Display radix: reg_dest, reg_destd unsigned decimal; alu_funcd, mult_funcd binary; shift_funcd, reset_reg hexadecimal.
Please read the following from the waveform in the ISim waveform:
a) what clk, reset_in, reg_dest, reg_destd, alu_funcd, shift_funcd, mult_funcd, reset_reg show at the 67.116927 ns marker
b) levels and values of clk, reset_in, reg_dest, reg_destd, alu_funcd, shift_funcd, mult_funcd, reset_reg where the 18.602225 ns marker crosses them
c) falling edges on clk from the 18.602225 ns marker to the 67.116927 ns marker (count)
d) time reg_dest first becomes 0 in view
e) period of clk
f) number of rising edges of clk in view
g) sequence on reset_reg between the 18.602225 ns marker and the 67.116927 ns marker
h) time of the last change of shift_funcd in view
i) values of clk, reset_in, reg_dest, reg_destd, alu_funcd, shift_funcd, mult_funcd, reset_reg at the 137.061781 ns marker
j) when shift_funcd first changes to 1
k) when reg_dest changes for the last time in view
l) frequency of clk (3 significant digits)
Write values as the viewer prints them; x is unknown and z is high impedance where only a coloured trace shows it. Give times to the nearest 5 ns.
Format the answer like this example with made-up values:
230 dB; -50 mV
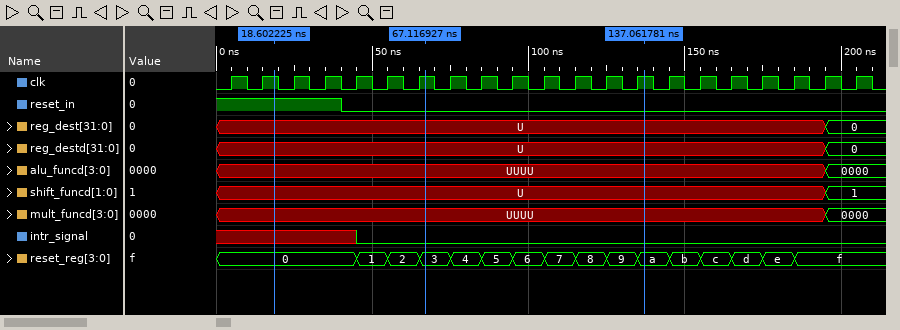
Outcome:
clk=1, reset_in=0, reg_dest=U, reg_destd=U, alu_funcd=UUUU, shift_funcd=U, mult_funcd=UUUU, reset_reg=3; clk=1, reset_in=1, reg_dest=U, reg_destd=U, alu_funcd=UUUU, shift_funcd=U, mult_funcd=UUUU, reset_reg=0; 5; 195 ns; 10 ns; 21; 0, 1, 2, 3; 195 ns; clk=1, reset_in=0, reg_dest=U, reg_destd=U, alu_funcd=UUUU, shift_funcd=U, mult_funcd=UUUU, reset_reg=a; 195 ns; 195 ns; 100 MHz
